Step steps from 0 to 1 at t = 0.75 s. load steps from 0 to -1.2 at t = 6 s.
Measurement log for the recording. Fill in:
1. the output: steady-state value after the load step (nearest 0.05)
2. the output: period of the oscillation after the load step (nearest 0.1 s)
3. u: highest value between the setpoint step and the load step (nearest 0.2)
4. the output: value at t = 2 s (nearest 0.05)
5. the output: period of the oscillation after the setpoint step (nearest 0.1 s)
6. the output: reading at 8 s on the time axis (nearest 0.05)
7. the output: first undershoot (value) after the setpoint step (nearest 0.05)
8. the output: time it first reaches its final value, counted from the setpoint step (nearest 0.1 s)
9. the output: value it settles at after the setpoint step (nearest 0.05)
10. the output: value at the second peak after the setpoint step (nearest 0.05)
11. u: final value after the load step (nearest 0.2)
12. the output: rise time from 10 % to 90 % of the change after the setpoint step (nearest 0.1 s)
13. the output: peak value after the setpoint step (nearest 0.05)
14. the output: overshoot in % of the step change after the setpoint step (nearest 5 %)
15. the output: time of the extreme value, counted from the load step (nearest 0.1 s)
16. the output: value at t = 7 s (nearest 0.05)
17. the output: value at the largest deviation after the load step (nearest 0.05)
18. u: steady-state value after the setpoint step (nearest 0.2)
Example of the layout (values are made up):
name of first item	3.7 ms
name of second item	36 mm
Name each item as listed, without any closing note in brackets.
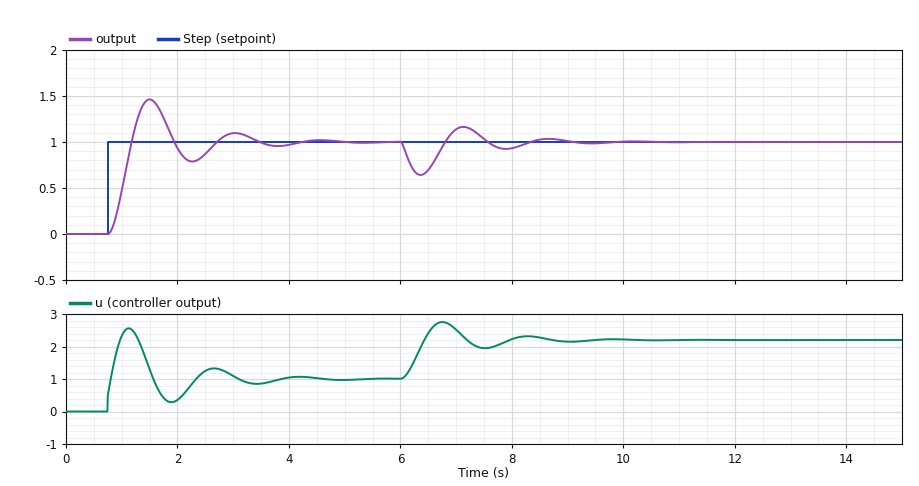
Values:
the output: steady-state value after the load step	1.00
the output: period of the oscillation after the load step	1.5 s
u: highest value between the setpoint step and the load step	2.6
the output: value at t = 2 s	0.95
the output: period of the oscillation after the setpoint step	1.5 s
the output: reading at 8 s on the time axis	0.95
the output: first undershoot (value) after the setpoint step	0.80
the output: time it first reaches its final value, counted from the setpoint step	0.4 s
the output: value it settles at after the setpoint step	1.00
the output: value at the second peak after the setpoint step	1.10
u: final value after the load step	2.2
the output: rise time from 10 % to 90 % of the change after the setpoint step	0.3 s
the output: peak value after the setpoint step	1.45
the output: overshoot in % of the step change after the setpoint step	45 %
the output: time of the extreme value, counted from the load step	0.4 s
the output: value at t = 7 s	1.15
the output: value at the largest deviation after the load step	0.65
u: steady-state value after the setpoint step	1.0
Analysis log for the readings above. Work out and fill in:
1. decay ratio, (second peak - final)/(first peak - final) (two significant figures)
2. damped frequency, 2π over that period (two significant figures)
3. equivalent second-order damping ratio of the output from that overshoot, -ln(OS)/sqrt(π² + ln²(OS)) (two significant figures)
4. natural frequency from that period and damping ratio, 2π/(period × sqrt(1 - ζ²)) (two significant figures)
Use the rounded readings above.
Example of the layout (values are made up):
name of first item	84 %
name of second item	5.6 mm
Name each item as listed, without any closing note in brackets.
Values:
decay ratio, (second peak - final)/(first peak - final)	0.22
damped frequency, 2π over that period	4.2 rad/s
equivalent second-order damping ratio of the output from that overshoot, -ln(OS)/sqrt(π² + ln²(OS))	0.25
natural frequency from that period and damping ratio, 2π/(period × sqrt(1 - ζ²))	4.3 rad/s
